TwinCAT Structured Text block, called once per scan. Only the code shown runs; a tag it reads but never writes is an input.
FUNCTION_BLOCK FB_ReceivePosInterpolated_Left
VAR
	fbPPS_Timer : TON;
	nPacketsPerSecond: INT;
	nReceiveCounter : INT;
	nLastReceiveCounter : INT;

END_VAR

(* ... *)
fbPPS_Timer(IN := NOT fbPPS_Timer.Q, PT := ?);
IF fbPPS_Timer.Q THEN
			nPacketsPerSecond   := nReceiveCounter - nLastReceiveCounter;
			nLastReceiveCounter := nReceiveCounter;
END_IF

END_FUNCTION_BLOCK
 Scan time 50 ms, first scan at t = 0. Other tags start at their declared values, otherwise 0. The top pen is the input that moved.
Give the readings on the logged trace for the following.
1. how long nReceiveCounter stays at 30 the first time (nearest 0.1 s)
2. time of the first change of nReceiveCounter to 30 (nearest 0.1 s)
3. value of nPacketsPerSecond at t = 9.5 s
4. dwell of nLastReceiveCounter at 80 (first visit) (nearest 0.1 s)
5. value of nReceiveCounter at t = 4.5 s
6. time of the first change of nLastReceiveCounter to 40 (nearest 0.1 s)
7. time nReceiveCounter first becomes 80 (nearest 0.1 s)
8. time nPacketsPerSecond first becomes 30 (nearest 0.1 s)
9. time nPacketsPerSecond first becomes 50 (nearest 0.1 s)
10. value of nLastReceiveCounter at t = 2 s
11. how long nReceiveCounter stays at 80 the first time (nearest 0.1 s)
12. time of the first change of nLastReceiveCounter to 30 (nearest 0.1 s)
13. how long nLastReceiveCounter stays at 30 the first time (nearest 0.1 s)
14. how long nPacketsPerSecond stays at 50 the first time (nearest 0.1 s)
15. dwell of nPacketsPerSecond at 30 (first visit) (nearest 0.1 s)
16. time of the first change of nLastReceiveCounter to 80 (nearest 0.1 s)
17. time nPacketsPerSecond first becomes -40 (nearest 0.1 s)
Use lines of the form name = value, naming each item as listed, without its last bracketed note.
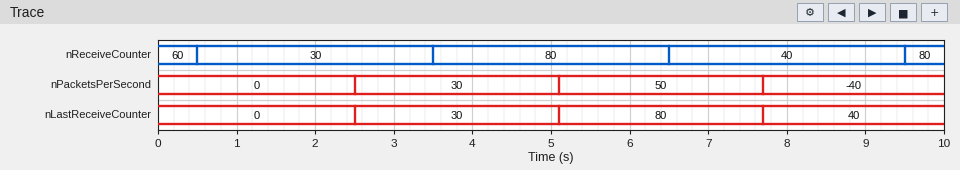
how long nReceiveCounter stays at 30 the first time = 3.0 s
time of the first change of nReceiveCounter to 30 = 0.5 s
value of nPacketsPerSecond at t = 9.5 s = -40
dwell of nLastReceiveCounter at 80 (first visit) = 2.6 s
value of nReceiveCounter at t = 4.5 s = 80
time of the first change of nLastReceiveCounter to 40 = 7.7 s
time nReceiveCounter first becomes 80 = 3.5 s
time nPacketsPerSecond first becomes 30 = 2.5 s
time nPacketsPerSecond first becomes 50 = 5.1 s
value of nLastReceiveCounter at t = 2 s = 0
how long nReceiveCounter stays at 80 the first time = 3.0 s
time of the first change of nLastReceiveCounter to 30 = 2.5 s
how long nLastReceiveCounter stays at 30 the first time = 2.6 s
how long nPacketsPerSecond stays at 50 the first time = 2.6 s
dwell of nPacketsPerSecond at 30 (first visit) = 2.6 s
time of the first change of nLastReceiveCounter to 80 = 5.1 s
time nPacketsPerSecond first becomes -40 = 7.7 s
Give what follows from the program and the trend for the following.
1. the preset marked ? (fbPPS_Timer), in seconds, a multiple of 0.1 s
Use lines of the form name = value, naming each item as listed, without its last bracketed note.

the preset marked ? (fbPPS_Timer), in seconds, a multiple of 0.1 s = 2.5 s
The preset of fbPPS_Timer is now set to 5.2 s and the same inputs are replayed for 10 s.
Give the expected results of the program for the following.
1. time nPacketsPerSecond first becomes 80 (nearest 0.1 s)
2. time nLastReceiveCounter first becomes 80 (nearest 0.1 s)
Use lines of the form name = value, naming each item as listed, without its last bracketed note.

time nPacketsPerSecond first becomes 80 = 5.2 s
time nLastReceiveCounter first becomes 80 = 5.2 s
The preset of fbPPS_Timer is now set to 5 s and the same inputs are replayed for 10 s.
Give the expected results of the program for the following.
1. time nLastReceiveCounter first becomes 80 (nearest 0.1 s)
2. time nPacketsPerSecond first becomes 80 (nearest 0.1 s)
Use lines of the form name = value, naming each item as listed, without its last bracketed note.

time nLastReceiveCounter first becomes 80 = 5.0 s
time nPacketsPerSecond first becomes 80 = 5.0 s
